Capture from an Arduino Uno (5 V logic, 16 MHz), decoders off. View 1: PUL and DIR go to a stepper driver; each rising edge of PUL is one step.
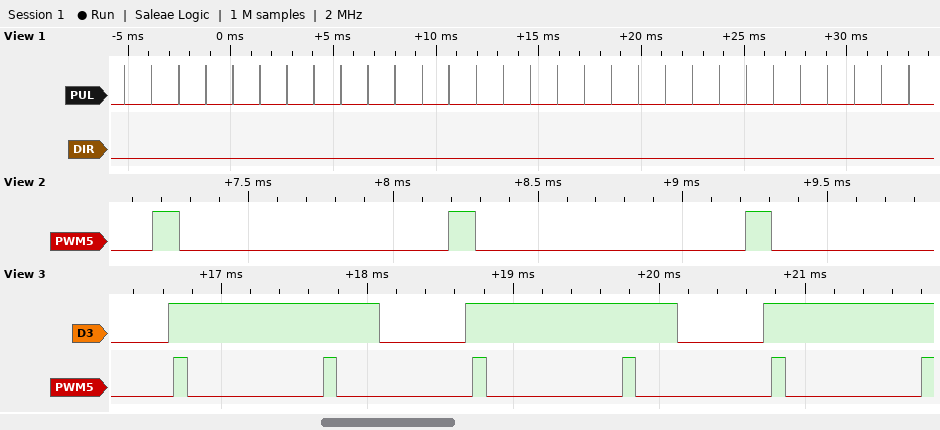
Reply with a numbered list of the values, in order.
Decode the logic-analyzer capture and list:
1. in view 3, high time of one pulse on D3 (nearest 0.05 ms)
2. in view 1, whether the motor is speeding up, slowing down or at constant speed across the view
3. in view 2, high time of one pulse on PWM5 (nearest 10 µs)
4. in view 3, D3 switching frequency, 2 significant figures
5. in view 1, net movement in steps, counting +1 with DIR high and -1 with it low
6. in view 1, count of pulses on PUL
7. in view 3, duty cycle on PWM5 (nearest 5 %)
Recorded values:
1. 1.45 ms
2. constant speed
3. 90 µs
4. 490 Hz
5. -30
6. 30
7. 10 %
